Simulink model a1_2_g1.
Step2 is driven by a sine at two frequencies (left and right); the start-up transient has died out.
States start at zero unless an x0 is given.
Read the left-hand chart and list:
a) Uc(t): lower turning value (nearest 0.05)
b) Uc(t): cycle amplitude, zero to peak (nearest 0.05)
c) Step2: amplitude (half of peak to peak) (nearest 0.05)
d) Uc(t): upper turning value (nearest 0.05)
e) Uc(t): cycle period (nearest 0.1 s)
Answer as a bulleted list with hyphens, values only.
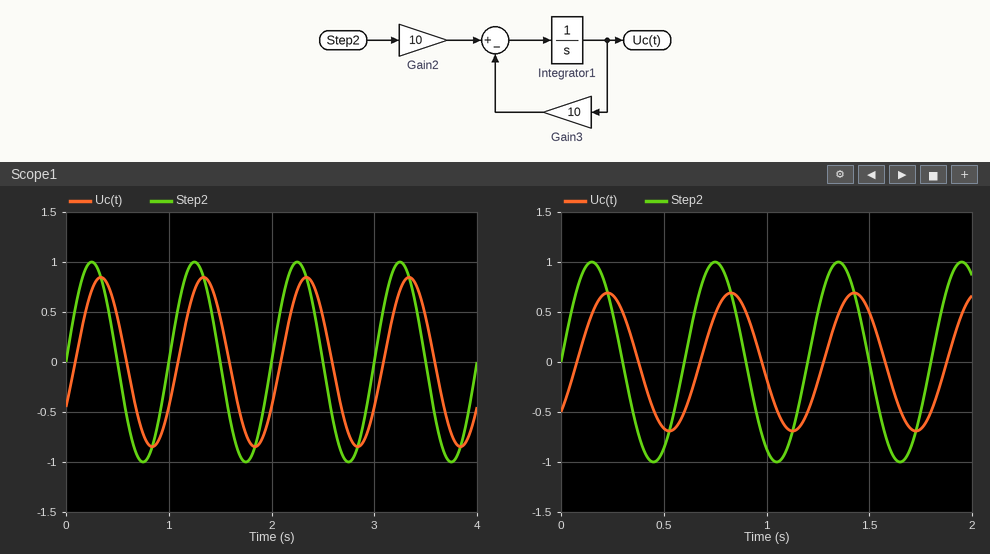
- -0.85
- 0.85
- 1.00
- 0.85
- 1.0 s
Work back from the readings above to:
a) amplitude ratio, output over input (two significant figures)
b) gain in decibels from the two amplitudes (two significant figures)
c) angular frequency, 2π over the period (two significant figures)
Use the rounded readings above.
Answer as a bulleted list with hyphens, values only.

- 0.85
- -1.4 dB
- 6.3 rad/s
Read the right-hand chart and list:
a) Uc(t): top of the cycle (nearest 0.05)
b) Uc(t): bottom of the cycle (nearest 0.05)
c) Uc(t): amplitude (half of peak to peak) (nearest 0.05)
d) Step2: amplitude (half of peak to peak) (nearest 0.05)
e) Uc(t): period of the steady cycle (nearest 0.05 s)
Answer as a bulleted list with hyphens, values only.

- 0.70
- -0.70
- 0.70
- 1.00
- 0.60 s
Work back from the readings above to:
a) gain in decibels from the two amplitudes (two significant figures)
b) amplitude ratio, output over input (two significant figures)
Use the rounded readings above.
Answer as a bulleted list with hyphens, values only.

- -3.1 dB
- 0.70
